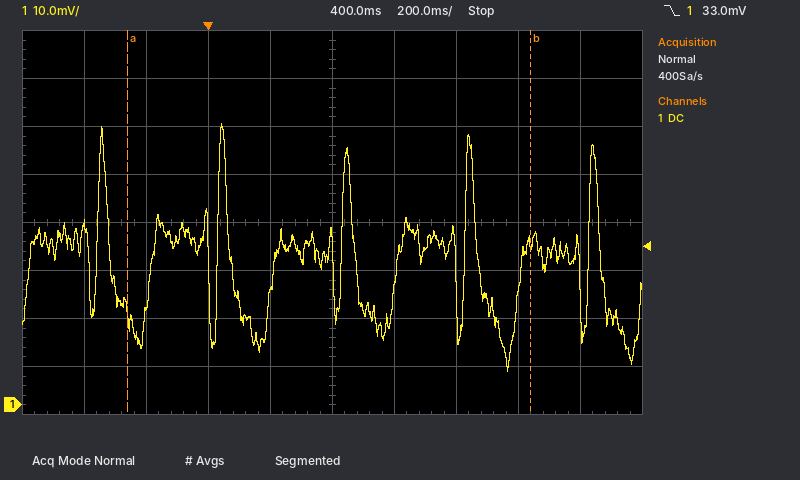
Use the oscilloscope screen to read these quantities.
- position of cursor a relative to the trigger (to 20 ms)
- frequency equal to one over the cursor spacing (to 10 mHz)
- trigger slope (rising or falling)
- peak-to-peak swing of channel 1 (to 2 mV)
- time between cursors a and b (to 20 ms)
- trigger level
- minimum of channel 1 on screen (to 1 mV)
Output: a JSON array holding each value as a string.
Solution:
["-260 ms", "770 mHz", "falling", "52 mV", "1.30 s", "33.0 mV", "7 mV"]
